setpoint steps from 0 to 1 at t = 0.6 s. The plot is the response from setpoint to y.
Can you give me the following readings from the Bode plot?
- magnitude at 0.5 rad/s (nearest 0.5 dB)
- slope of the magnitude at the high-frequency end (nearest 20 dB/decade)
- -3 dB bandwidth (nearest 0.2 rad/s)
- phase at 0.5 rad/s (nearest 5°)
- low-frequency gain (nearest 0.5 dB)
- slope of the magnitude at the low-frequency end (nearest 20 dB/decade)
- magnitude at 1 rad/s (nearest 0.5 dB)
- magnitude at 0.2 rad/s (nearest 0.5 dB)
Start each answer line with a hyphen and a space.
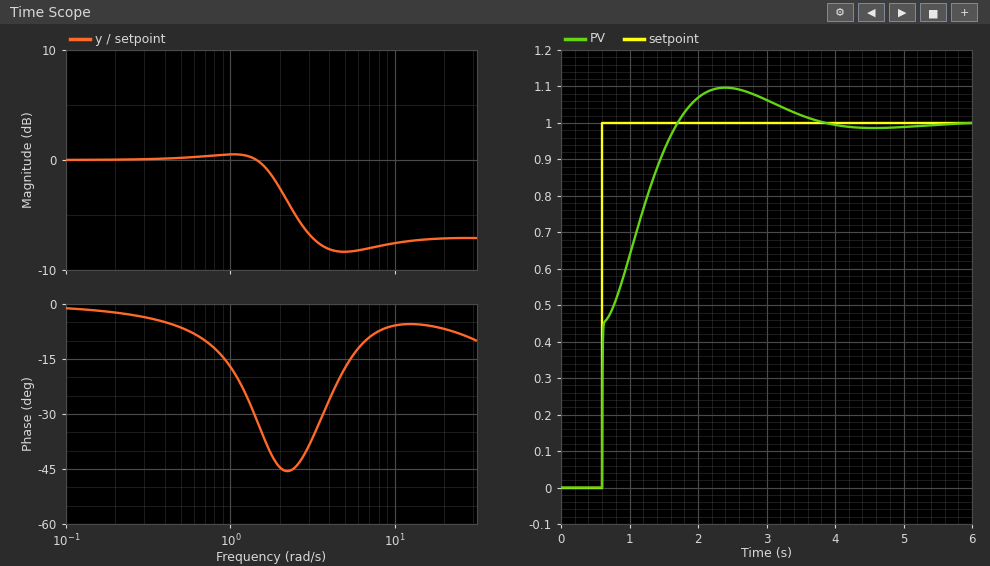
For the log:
- 0.0 dB
- 0 dB/decade
- 2.0 rad/s
- -5°
- 0.0 dB
- 0 dB/decade
- 0.5 dB
- 0.0 dB
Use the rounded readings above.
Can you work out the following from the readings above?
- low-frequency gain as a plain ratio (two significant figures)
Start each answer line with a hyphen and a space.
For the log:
- 1.0
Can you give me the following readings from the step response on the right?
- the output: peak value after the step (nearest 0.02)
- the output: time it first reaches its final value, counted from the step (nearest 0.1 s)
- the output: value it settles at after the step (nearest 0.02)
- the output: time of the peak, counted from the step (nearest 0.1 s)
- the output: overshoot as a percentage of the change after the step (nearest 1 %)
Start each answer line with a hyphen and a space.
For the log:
- 1.10
- 1.1 s
- 1.00
- 1.8 s
- 10 %
